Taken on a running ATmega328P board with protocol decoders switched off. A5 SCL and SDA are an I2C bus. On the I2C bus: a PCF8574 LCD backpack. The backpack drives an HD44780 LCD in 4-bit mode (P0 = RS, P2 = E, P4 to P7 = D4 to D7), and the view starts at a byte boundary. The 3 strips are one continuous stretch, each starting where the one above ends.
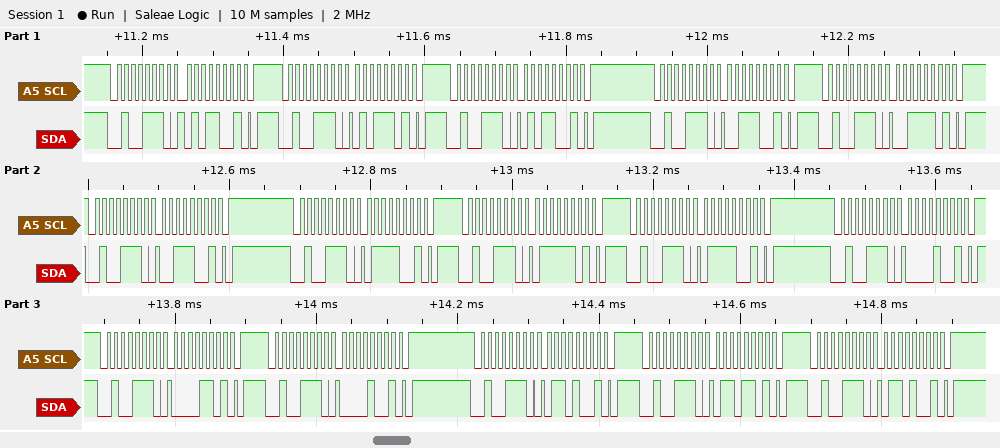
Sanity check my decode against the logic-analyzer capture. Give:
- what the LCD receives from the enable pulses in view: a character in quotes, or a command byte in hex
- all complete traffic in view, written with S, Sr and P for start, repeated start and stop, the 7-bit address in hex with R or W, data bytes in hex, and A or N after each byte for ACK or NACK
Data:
'S' 'p'
S 27W A 59 A P S 27W A 5D A P S 27W A 59 A P S 27W A 39 A P S 27W A 3D A P S 27W A 39 A P S 27W A 79 A P S 27W A 7D A P S 27W A 79 A P S 27W A 09 A P S 27W A 0D A P S 27W A 09 A P S 27W A 69 A P S 27W A 6D A P S 27W A 69 A P
